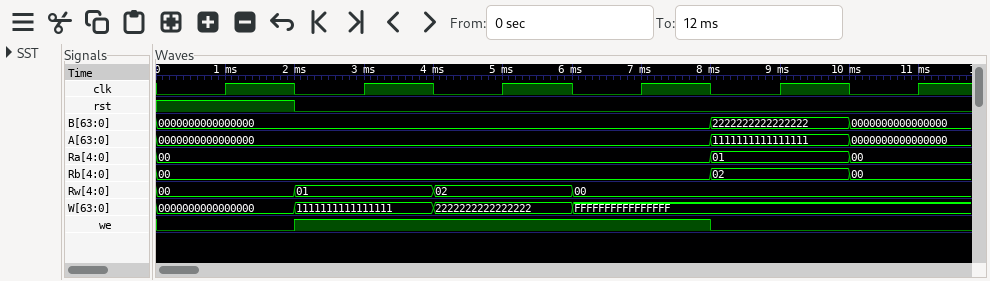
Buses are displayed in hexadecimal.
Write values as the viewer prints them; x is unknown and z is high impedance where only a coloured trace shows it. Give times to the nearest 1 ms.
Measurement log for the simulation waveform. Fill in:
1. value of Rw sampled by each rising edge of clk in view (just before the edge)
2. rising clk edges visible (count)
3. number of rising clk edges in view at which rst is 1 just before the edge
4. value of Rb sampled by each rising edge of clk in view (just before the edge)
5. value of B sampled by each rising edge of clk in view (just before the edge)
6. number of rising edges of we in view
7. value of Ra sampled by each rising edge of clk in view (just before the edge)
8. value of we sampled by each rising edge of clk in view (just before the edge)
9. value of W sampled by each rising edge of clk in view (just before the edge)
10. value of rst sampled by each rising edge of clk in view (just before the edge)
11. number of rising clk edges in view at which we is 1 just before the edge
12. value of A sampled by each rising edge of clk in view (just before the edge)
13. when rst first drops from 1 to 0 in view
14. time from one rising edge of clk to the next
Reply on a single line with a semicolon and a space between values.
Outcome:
00, 01, 02, 00, 00, 00; 6; 1; 00, 00, 00, 00, 02, 00; 0000000000000000, 0000000000000000, 0000000000000000, 0000000000000000, 2222222222222222, 0000000000000000; 1; 00, 00, 00, 00, 01, 00; 0 1 1 1 0 0; 0000000000000000, 1111111111111111, 2222222222222222, FFFFFFFFFFFFFFFF, FFFFFFFFFFFFFFFF, FFFFFFFFFFFFFFFF; 1 0 0 0 0 0; 3; 0000000000000000, 0000000000000000, 0000000000000000, 0000000000000000, 1111111111111111, 0000000000000000; 2 ms; 2 ms
